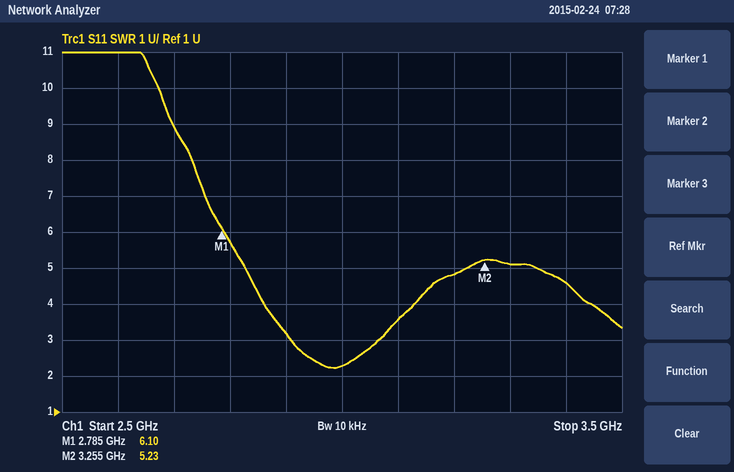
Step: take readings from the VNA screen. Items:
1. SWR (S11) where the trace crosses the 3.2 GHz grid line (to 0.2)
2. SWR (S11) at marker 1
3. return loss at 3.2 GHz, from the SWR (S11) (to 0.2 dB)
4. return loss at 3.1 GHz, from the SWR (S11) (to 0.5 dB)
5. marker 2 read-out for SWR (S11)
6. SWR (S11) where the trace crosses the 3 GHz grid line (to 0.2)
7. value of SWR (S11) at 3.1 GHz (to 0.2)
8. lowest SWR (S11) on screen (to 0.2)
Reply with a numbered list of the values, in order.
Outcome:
1. 4.8
2. 6.10
3. 3.6 dB
4. 5.0 dB
5. 5.23
6. 2.2
7. 3.6
8. 2.2
